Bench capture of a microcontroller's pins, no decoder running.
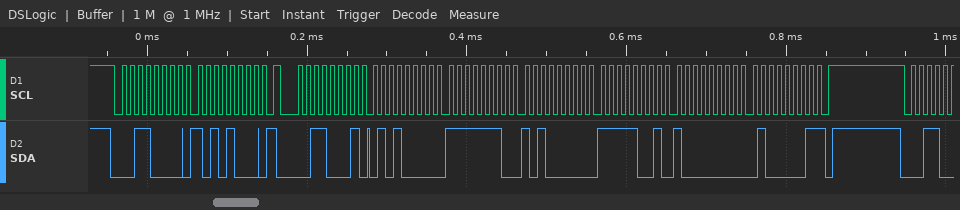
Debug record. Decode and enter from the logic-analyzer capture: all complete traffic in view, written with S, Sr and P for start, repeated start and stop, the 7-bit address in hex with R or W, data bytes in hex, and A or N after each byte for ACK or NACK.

S 18W A A8 A Sr 18R A 50 A FE A A0 A F9 A 80 A 41 N P
